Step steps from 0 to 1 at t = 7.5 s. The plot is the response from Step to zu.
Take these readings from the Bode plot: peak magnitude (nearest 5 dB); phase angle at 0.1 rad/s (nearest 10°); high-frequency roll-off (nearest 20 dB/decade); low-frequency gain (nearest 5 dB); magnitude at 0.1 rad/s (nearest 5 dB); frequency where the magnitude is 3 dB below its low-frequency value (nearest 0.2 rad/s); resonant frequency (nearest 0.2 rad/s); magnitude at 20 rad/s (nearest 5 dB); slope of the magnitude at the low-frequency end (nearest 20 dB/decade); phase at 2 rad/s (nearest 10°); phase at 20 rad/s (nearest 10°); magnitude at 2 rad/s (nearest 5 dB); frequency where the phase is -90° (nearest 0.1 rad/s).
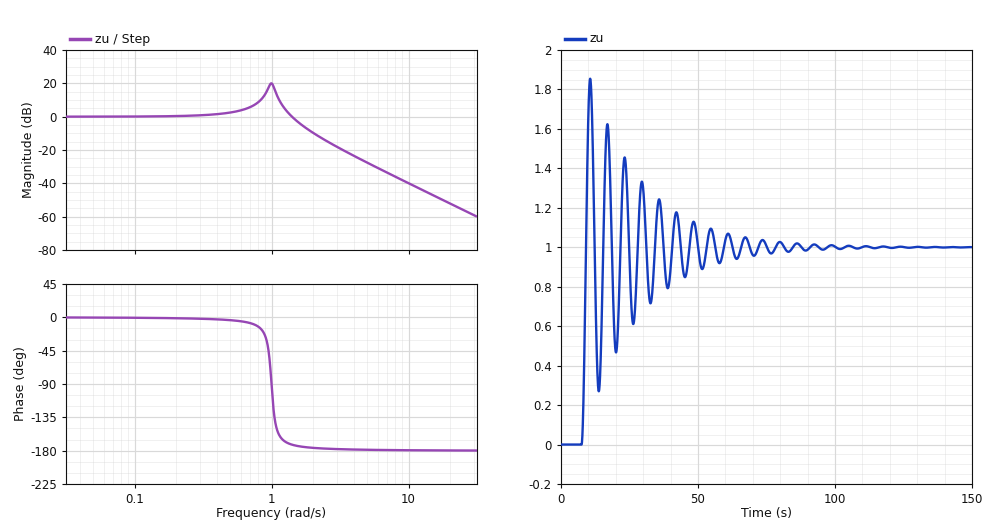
20 dB
0°
-40 dB/decade
0 dB
0 dB
1.6 rad/s
1.0 rad/s
-50 dB
0 dB/decade
-180°
-180°
-10 dB
1.0 rad/s
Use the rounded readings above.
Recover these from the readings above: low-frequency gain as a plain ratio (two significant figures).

1.0
